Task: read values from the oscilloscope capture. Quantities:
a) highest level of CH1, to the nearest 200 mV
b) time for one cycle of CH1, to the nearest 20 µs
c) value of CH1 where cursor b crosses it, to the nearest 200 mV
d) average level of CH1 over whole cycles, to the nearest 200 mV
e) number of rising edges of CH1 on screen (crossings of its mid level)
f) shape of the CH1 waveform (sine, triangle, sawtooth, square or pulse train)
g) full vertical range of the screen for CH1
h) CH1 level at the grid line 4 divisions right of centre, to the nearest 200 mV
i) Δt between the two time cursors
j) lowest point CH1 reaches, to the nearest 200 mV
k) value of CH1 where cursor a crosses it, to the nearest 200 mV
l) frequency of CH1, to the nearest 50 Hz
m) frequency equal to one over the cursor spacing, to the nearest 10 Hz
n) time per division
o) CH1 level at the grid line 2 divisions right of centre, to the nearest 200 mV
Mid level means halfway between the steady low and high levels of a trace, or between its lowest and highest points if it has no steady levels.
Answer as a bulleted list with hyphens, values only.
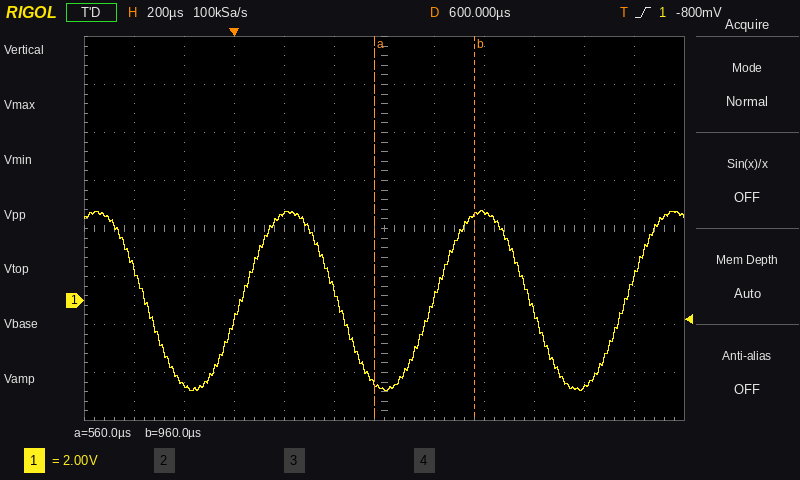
- 3.8 V
- 760 µs
- 3.6 V
- 0.0 V
- 3
- sine
- 16 V
- -3.6 V
- 400 µs
- -3.8 V
- -3.4 V
- 1.30 kHz
- 2.50 kHz
- 200 µs
- 3.6 V
